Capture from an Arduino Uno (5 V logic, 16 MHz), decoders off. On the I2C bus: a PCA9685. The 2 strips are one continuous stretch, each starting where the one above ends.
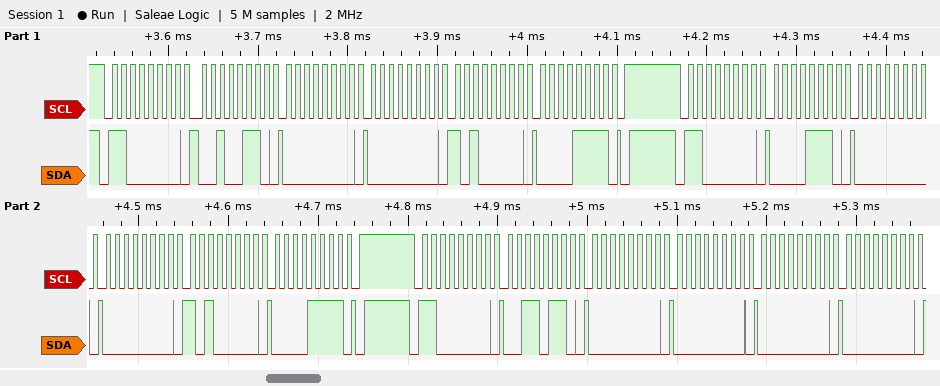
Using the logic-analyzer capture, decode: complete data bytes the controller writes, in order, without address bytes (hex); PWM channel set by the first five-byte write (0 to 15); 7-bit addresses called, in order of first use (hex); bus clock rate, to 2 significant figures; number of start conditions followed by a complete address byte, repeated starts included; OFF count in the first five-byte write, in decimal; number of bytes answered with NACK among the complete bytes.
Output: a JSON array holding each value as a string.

["26 00 00 A0 0F 0E 00 00 A0 0F 36 00 00 00 00", "8", "0x60", "100 kHz", "3", "4000", "0"]
